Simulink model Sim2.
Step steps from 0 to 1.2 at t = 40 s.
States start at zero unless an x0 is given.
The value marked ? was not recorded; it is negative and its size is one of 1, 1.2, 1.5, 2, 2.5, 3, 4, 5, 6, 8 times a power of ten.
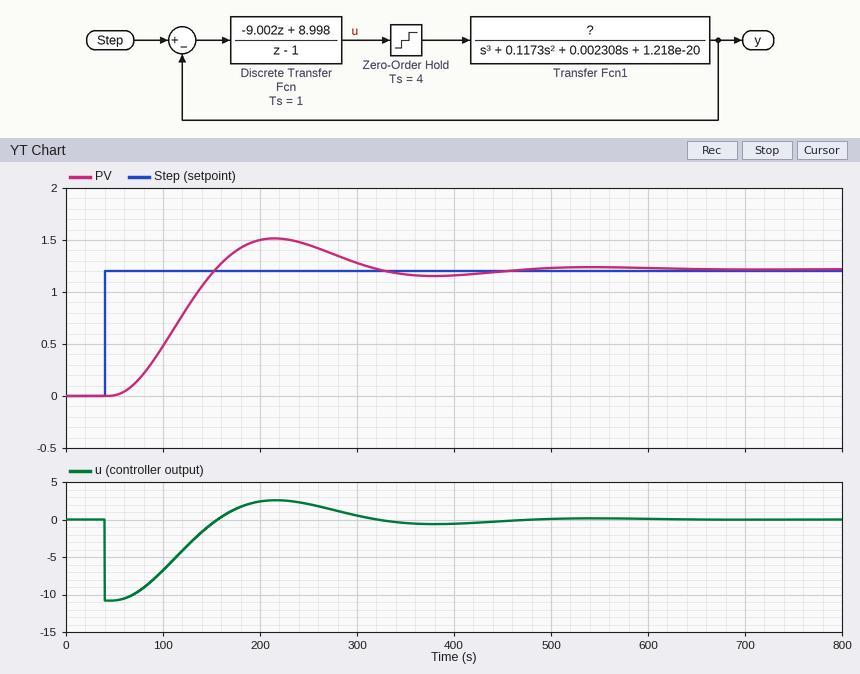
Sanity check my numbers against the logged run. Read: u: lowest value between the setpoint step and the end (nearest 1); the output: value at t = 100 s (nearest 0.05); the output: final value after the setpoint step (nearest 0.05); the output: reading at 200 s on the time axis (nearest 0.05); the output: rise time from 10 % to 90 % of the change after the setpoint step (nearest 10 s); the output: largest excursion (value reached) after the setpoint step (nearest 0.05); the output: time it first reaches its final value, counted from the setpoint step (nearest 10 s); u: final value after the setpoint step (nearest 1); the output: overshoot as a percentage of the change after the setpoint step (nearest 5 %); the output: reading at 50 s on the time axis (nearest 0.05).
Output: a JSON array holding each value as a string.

["-11", "0.50", "1.20", "1.50", "70 s", "1.50", "110 s", "0", "25 %", "0.00"]
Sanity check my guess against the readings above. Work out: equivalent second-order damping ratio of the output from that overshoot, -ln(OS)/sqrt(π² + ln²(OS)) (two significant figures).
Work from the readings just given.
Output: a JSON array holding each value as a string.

["0.40"]
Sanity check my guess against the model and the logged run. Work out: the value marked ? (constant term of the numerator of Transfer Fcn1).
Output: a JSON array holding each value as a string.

["-5e-06"]
